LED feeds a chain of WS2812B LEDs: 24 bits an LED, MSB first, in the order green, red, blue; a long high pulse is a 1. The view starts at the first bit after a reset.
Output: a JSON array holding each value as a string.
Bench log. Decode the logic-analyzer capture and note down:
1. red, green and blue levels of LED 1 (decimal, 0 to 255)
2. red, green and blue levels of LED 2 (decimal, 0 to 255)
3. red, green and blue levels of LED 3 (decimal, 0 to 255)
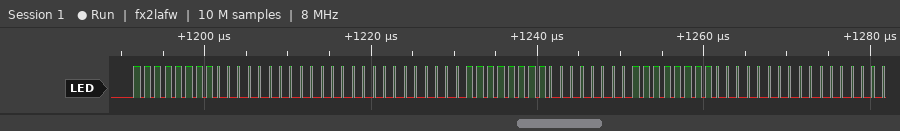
["0, 255, 0", "255, 0, 0", "0, 255, 0"]
